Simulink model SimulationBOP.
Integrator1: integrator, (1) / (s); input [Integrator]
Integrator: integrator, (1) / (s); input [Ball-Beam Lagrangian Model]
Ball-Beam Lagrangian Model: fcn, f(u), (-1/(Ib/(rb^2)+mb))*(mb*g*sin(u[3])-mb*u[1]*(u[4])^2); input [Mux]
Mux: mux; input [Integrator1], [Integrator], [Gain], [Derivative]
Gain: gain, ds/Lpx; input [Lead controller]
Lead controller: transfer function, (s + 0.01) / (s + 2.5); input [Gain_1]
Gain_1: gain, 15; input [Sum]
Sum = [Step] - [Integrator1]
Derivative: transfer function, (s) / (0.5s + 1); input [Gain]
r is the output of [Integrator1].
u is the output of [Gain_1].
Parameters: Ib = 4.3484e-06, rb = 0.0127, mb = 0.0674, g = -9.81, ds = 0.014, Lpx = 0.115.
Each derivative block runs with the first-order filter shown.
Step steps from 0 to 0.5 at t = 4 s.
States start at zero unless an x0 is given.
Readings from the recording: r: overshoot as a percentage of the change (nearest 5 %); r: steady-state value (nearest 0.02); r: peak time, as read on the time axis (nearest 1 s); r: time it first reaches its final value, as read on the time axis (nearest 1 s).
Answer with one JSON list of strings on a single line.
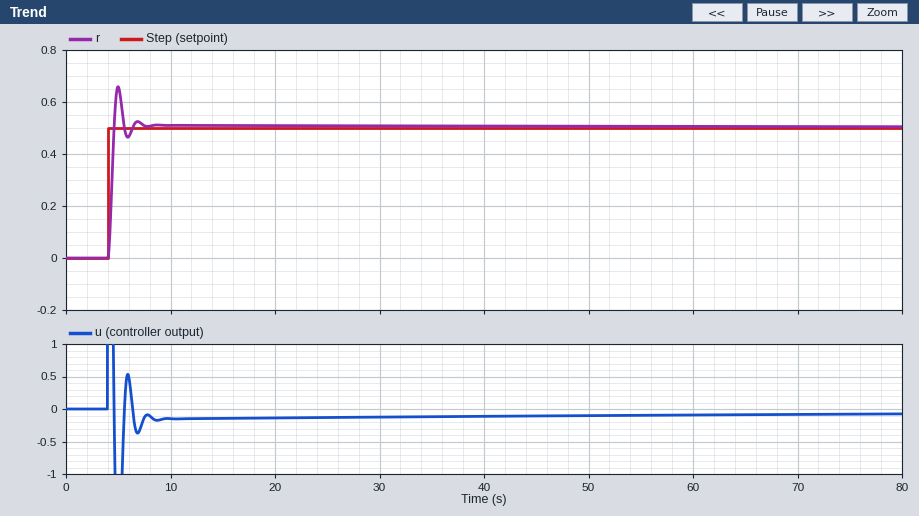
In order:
["30 %", "0.50", "5 s", "5 s"]
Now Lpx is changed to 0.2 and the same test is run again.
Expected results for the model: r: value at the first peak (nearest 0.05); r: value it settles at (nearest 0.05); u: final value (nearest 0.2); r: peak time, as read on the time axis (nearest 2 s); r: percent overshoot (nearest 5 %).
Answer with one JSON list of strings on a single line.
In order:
["0.60", "0.50", "0.0", "6 s", "20 %"]
